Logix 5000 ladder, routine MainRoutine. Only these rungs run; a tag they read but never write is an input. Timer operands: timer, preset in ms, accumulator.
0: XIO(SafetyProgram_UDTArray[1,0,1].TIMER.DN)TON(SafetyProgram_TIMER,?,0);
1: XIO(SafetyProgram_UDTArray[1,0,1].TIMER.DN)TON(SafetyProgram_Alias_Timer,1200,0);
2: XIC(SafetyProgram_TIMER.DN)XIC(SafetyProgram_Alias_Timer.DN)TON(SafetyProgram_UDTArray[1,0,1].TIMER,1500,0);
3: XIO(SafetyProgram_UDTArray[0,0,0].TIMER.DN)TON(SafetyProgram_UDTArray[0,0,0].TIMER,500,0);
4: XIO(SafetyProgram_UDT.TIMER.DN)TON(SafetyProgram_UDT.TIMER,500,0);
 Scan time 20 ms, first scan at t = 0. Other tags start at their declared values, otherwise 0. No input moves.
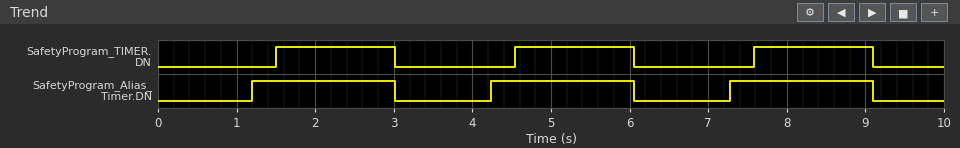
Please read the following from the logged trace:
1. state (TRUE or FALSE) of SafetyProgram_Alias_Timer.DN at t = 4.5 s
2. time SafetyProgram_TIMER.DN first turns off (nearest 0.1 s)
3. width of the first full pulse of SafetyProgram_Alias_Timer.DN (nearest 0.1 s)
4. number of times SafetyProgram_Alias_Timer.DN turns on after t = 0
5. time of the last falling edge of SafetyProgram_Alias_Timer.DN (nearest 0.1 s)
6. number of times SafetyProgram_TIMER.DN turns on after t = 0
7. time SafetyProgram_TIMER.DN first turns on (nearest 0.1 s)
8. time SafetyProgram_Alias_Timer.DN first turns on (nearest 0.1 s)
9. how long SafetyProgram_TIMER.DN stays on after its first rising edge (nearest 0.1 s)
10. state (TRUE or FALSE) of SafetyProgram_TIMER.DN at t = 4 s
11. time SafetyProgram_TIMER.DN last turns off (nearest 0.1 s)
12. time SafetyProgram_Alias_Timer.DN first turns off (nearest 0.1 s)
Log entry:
TRUE
3.0 s
1.8 s
3
9.1 s
3
1.5 s
1.2 s
1.5 s
FALSE
9.1 s
3.0 s
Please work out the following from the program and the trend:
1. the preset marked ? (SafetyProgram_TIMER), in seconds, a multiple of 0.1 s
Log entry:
1.5 s
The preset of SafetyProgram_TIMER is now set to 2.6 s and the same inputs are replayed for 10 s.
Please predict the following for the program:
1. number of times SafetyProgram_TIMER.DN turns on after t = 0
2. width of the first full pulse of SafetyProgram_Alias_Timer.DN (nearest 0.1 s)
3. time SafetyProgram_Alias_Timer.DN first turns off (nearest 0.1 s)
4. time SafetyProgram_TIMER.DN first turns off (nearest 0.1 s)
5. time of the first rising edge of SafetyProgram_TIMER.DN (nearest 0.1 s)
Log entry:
2
2.9 s
4.1 s
4.1 s
2.6 s
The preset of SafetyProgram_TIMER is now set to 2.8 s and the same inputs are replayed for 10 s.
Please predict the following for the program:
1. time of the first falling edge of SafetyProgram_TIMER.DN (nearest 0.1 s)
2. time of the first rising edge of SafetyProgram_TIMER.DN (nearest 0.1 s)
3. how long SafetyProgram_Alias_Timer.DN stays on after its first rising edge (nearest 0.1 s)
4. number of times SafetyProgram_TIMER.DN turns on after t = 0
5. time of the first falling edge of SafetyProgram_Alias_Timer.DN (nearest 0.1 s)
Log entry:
4.3 s
2.8 s
3.1 s
2
4.3 s
